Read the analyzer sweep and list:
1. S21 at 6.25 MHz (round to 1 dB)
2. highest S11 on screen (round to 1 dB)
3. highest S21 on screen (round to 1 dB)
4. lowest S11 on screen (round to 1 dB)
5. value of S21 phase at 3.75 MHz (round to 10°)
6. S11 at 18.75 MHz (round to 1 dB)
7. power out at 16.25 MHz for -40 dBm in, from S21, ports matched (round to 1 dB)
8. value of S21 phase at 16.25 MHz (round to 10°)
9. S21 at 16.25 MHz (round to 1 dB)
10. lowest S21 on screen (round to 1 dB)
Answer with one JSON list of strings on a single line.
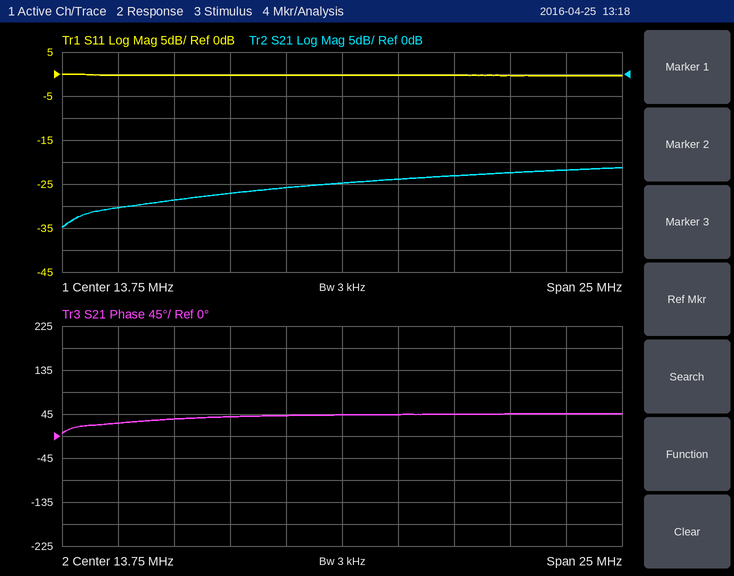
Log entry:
["-29 dB", "0 dB", "-21 dB", "0 dB", "30°", "0 dB", "-64 dBm", "40°", "-24 dB", "-35 dB"]
